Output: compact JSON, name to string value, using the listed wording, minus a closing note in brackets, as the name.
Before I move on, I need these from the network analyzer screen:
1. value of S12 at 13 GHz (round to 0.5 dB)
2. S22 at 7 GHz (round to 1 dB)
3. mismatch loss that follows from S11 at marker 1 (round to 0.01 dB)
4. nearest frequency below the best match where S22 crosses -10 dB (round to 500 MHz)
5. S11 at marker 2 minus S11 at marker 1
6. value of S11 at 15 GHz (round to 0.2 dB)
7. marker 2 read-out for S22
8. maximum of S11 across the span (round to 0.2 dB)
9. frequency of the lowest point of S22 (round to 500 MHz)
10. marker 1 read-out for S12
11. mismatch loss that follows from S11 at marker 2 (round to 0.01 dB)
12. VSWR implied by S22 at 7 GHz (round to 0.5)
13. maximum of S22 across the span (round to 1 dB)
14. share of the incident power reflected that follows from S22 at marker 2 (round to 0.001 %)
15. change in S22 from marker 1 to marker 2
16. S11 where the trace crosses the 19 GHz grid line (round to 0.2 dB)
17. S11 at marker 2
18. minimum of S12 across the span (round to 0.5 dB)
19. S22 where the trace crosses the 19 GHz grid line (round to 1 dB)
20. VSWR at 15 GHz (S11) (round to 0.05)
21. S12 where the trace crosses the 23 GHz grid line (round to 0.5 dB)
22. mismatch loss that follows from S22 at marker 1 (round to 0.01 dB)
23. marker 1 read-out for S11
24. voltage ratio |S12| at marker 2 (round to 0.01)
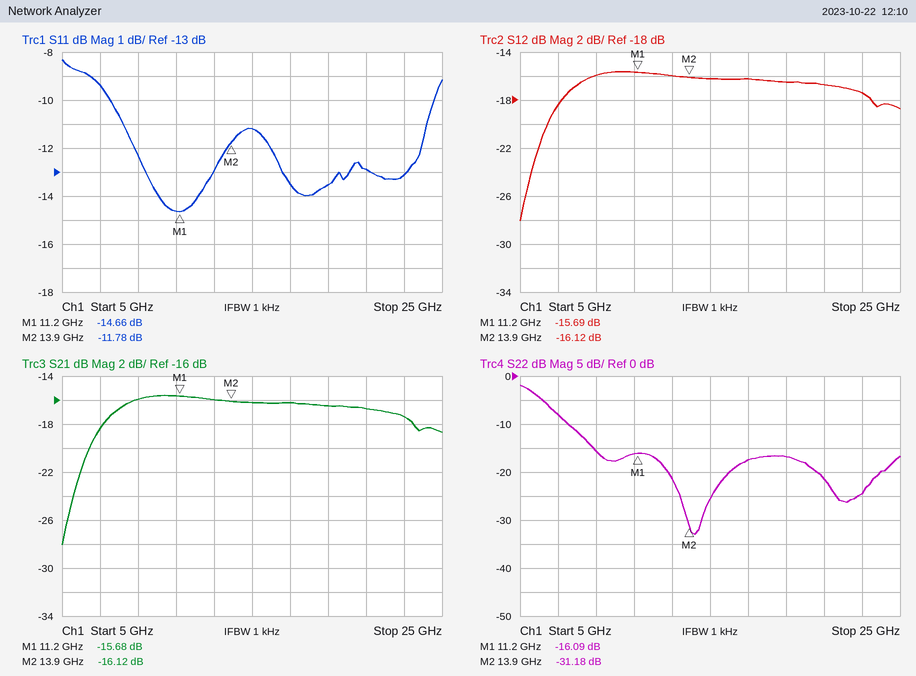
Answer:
{"value of S12 at 13 GHz": "-16.0 dB", "S22 at 7 GHz": "-8 dB", "mismatch loss that follows from S11 at marker 1": "0.15 dB", "nearest frequency below the best match where S22 crosses -10 dB": "7.5 GHz", "S11 at marker 2 minus S11 at marker 1": "2.88 dB", "value of S11 at 15 GHz": "-11.2 dB", "marker 2 read-out for S22": "-31.18 dB", "maximum of S11 across the span": "-8.4 dB", "frequency of the lowest point of S22": "14.0 GHz", "marker 1 read-out for S12": "-15.69 dB", "mismatch loss that follows from S11 at marker 2": "0.30 dB", "VSWR implied by S22 at 7 GHz": "2.5", "maximum of S22 across the span": "-2 dB", "share of the incident power reflected that follows from S22 at marker 2": "0.076 %", "change in S22 from marker 1 to marker 2": "-15.09 dB", "S11 where the trace crosses the 19 GHz grid line": "-13.6 dB", "S11 at marker 2": "-11.78 dB", "minimum of S12 across the span": "-28.0 dB", "S22 where the trace crosses the 19 GHz grid line": "-17 dB", "VSWR at 15 GHz (S11)": "1.75", "S12 where the trace crosses the 23 GHz grid line": "-17.5 dB", "mismatch loss that follows from S22 at marker 1": "0.11 dB", "marker 1 read-out for S11": "-14.66 dB", "voltage ratio |S12| at marker 2": "0.16"}
